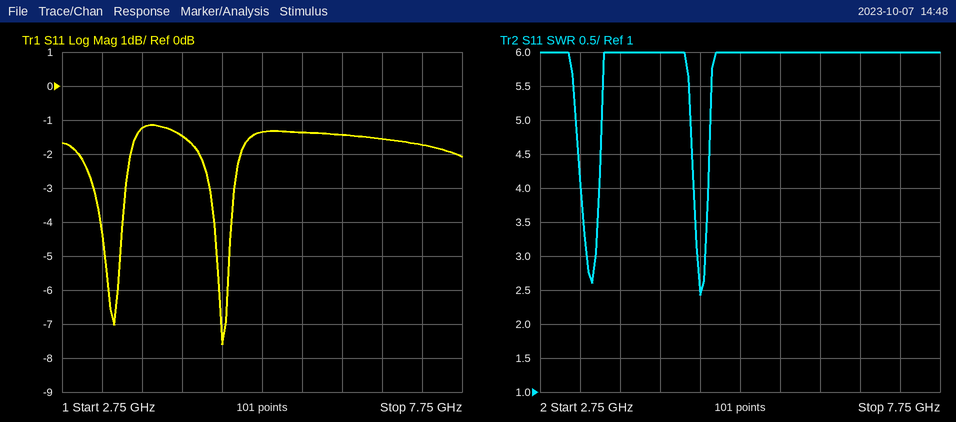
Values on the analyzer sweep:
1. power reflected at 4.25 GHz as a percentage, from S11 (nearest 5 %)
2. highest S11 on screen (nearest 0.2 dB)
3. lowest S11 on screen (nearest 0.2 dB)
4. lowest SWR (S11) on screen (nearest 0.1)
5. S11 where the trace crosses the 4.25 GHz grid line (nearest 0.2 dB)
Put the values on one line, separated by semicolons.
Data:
70 %; -1.2 dB; -7.6 dB; 2.4; -1.4 dB
